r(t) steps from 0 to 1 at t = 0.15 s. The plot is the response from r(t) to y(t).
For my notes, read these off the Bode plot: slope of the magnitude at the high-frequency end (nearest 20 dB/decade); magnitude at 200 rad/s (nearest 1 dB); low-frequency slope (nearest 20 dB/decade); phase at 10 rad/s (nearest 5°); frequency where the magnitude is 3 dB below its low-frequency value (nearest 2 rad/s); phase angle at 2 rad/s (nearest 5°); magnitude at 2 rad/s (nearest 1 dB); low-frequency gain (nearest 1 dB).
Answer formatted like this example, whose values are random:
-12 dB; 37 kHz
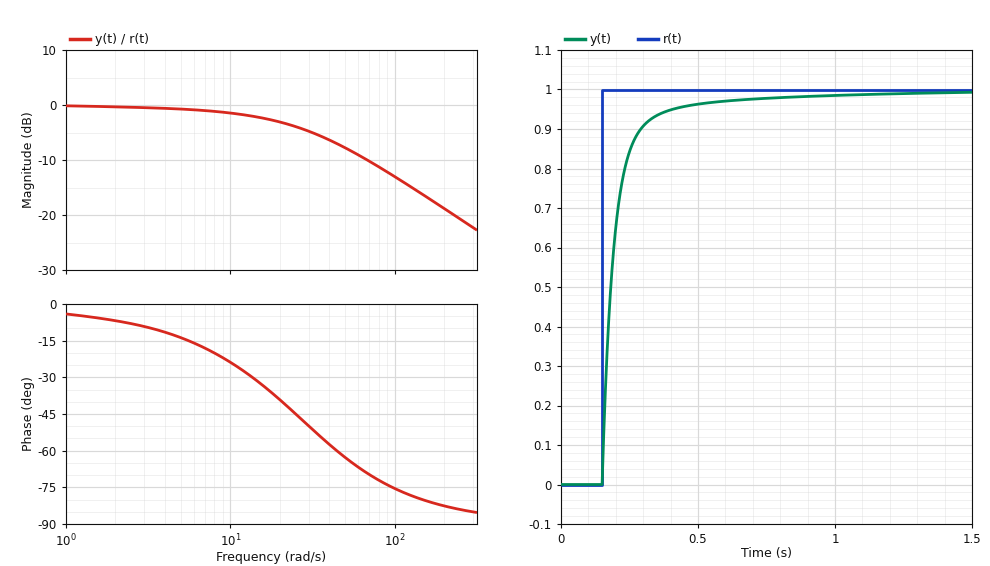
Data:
-20 dB/decade; -19 dB; 0 dB/decade; -25°; 20 rad/s; -5°; 0 dB; 0 dB
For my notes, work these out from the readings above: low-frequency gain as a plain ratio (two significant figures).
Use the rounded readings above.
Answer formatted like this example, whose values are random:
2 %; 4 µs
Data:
1.0
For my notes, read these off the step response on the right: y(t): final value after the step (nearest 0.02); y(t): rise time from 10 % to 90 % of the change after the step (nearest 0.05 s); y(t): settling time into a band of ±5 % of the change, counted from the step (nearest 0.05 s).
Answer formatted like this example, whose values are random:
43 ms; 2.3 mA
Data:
1.00; 0.15 s; 0.25 s
